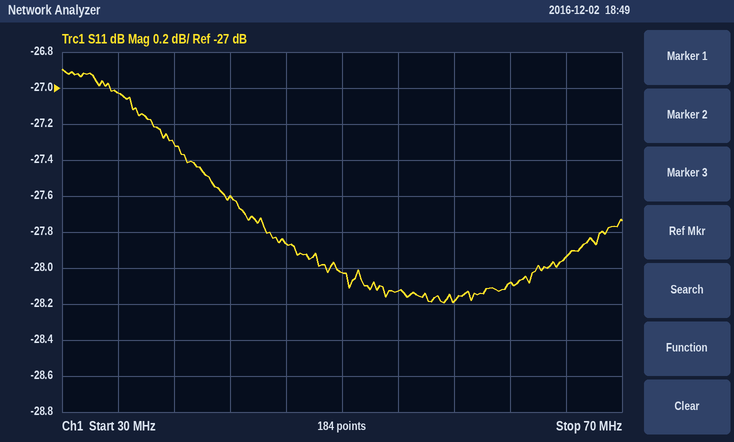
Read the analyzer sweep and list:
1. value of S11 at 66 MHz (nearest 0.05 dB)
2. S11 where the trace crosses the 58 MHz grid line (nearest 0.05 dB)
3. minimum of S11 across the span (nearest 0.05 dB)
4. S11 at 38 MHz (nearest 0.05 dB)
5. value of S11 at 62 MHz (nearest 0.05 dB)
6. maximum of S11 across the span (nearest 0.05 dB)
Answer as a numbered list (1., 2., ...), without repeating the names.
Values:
1. -27.95 dB
2. -28.20 dB
3. -28.20 dB
4. -27.30 dB
5. -28.10 dB
6. -26.90 dB
